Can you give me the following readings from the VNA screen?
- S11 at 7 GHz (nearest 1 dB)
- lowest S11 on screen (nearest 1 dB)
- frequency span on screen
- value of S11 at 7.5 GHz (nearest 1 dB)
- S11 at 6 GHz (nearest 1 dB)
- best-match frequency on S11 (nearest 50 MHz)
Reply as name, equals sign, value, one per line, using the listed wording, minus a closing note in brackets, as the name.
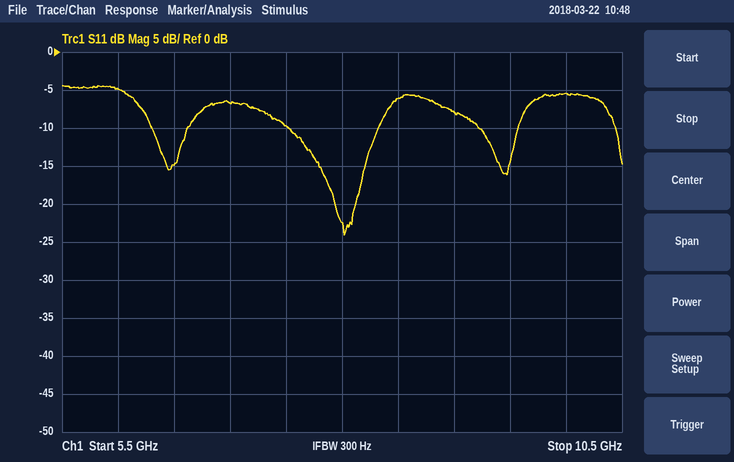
S11 at 7 GHz = -7 dB
lowest S11 on screen = -24 dB
frequency span on screen = 5 GHz
value of S11 at 7.5 GHz = -10 dB
S11 at 6 GHz = -5 dB
best-match frequency on S11 = 8.00 GHz
